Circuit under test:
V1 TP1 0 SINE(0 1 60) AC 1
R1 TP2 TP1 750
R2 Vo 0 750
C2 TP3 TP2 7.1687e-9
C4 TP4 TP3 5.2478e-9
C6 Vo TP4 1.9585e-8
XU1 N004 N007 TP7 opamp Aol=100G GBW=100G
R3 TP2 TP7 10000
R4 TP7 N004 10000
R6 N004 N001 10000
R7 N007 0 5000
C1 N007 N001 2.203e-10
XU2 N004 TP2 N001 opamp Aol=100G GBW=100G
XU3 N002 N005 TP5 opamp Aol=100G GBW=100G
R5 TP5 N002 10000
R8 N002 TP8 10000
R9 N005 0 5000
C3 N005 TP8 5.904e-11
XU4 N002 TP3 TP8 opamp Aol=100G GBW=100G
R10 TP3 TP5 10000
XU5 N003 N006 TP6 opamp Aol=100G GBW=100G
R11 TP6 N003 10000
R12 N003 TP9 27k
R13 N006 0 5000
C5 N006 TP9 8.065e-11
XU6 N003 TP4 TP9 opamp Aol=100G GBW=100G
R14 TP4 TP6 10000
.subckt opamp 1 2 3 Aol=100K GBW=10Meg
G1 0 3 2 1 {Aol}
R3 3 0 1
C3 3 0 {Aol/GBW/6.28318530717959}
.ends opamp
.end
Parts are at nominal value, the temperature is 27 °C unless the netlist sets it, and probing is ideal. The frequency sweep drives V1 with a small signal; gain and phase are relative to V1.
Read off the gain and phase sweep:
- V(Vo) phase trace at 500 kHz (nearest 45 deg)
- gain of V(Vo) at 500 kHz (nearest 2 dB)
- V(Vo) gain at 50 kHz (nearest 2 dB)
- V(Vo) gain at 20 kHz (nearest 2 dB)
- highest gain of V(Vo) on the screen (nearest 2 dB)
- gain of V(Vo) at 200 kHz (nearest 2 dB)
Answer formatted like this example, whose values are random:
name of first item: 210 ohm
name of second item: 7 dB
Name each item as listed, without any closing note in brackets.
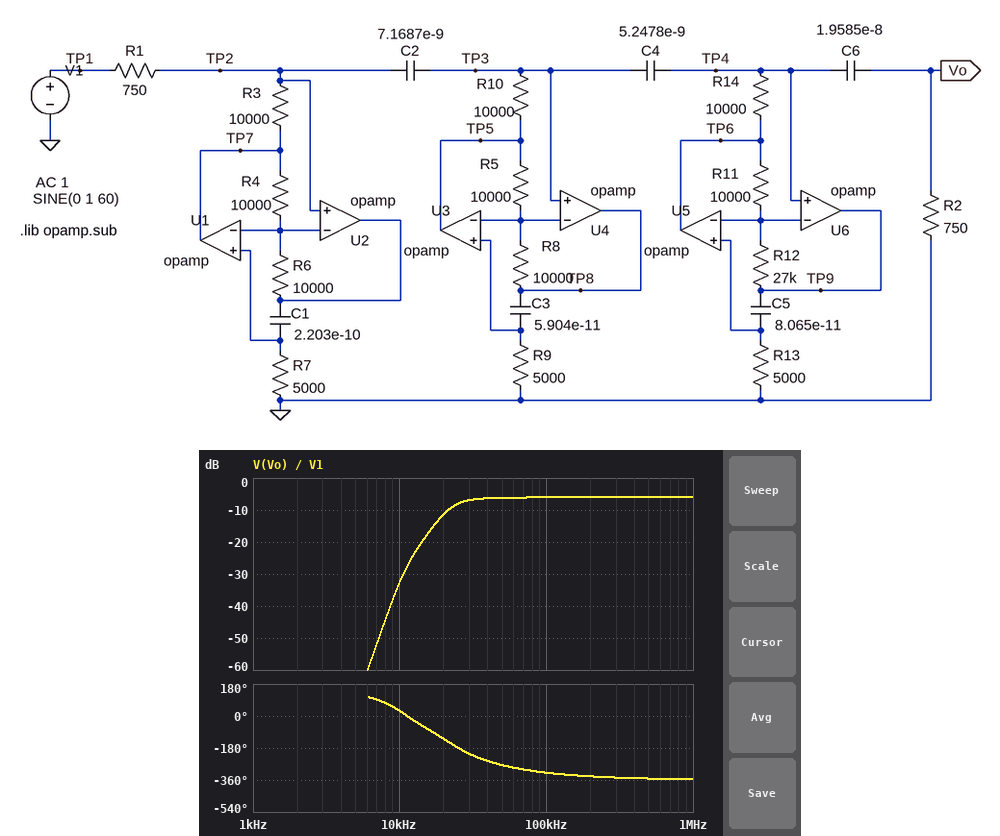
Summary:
V(Vo) phase trace at 500 kHz: -360 deg
gain of V(Vo) at 500 kHz: -6 dB
V(Vo) gain at 50 kHz: -6 dB
V(Vo) gain at 20 kHz: -12 dB
highest gain of V(Vo) on the screen: -6 dB
gain of V(Vo) at 200 kHz: -6 dB
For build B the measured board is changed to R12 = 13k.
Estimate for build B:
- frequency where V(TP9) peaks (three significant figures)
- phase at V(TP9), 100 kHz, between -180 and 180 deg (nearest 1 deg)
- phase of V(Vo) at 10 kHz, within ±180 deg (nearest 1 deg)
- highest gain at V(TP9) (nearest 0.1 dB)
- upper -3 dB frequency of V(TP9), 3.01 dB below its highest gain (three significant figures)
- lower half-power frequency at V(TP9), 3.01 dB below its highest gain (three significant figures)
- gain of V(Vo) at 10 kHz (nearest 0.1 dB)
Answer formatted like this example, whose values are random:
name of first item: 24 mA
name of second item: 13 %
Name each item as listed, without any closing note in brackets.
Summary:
frequency where V(TP9) peaks: 23.0 kHz
phase at V(TP9), 100 kHz, between -180 and 180 deg: -37 deg
phase of V(Vo) at 10 kHz, within ±180 deg: 66 deg
highest gain at V(TP9): 18.1 dB
upper -3 dB frequency of V(TP9), 3.01 dB below its highest gain: 36.0 kHz
lower half-power frequency at V(TP9), 3.01 dB below its highest gain: 17.8 kHz
gain of V(Vo) at 10 kHz: -41.5 dB
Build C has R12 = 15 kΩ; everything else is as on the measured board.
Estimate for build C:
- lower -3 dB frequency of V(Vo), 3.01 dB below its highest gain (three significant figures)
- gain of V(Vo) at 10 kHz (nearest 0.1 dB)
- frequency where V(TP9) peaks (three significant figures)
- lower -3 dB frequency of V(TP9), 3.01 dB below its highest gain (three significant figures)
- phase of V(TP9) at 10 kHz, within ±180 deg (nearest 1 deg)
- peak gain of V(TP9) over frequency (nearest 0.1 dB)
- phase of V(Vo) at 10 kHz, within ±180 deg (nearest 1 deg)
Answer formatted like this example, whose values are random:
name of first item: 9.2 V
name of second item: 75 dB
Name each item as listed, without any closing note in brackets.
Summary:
lower -3 dB frequency of V(Vo), 3.01 dB below its highest gain: 20.9 kHz
gain of V(Vo) at 10 kHz: -39.7 dB
frequency where V(TP9) peaks: 23.0 kHz
lower -3 dB frequency of V(TP9), 3.01 dB below its highest gain: 17.3 kHz
phase of V(TP9) at 10 kHz, within ±180 deg: -74 deg
peak gain of V(TP9) over frequency: 17.8 dB
phase of V(Vo) at 10 kHz, within ±180 deg: 62 deg
